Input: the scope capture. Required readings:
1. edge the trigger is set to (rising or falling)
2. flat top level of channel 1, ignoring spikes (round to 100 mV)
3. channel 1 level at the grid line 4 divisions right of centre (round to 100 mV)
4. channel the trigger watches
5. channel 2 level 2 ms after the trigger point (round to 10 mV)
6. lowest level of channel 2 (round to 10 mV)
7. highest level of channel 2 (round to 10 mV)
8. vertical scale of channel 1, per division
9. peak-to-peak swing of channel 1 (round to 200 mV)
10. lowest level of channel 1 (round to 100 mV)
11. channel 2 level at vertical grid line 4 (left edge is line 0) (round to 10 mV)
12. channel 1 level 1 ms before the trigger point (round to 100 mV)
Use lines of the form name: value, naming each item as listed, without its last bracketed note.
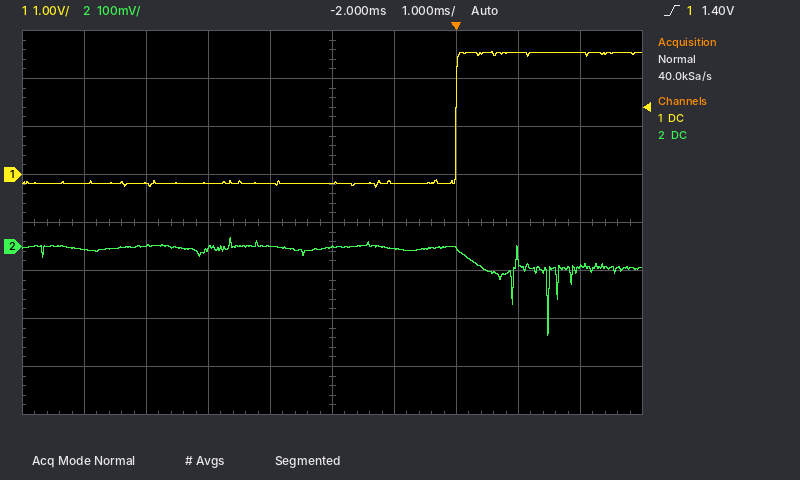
edge the trigger is set to: rising
flat top level of channel 1, ignoring spikes: 2.5 V
channel 1 level at the grid line 4 divisions right of centre: 2.5 V
channel the trigger watches: channel 1
channel 2 level 2 ms after the trigger point: -40 mV
lowest level of channel 2: -190 mV
highest level of channel 2: 20 mV
vertical scale of channel 1, per division: 1 V
peak-to-peak swing of channel 1: 2.8 V
lowest level of channel 1: -300 mV
channel 2 level at vertical grid line 4 (left edge is line 0): 0 mV
channel 1 level 1 ms before the trigger point: -200 mV
